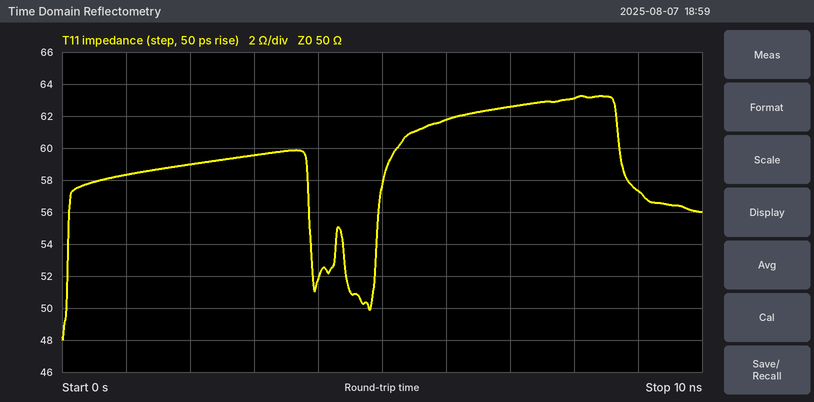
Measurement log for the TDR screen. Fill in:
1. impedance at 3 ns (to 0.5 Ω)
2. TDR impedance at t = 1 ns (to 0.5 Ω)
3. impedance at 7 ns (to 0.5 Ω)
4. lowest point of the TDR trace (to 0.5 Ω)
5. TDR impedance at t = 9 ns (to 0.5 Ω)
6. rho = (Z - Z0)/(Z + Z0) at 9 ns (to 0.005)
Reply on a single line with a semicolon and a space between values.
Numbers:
59.5 Ω; 58.5 Ω; 62.5 Ω; 48.0 Ω; 57.5 Ω; +0.070
